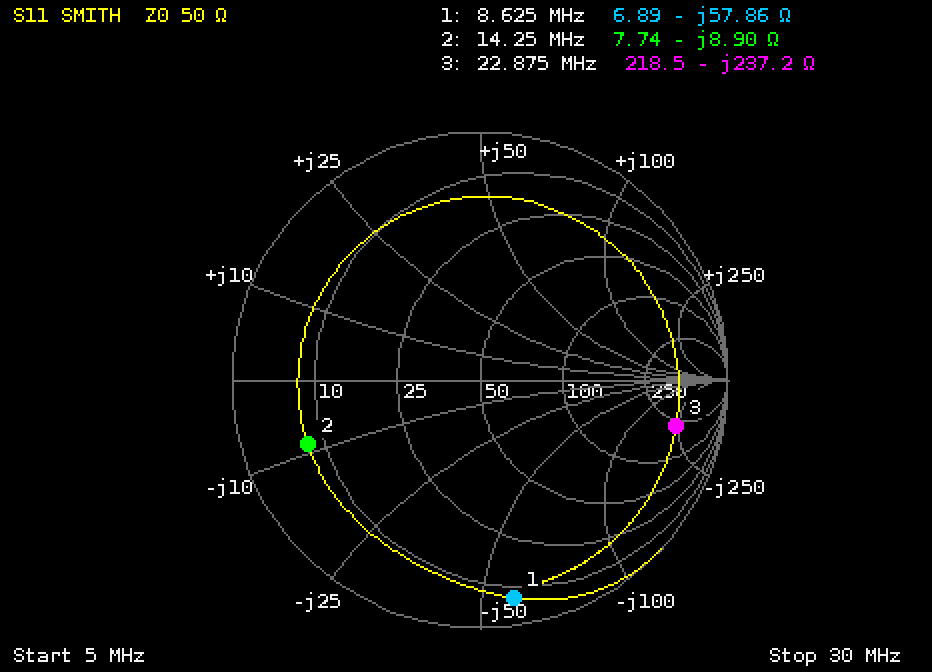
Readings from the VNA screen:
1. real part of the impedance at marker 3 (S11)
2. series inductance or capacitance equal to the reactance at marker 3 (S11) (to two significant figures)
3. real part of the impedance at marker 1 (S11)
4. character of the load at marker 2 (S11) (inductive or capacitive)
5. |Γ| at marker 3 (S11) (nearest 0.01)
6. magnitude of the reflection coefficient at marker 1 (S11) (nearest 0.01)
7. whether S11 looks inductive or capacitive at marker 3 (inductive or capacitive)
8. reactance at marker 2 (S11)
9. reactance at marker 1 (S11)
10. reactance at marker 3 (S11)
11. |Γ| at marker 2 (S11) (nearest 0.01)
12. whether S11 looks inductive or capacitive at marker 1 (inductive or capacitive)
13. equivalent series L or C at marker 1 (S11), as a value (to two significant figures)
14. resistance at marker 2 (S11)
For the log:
218.5 Ω
29 pF
6.89 Ω
capacitive
0.81
0.89
capacitive
-8.90 Ω
-57.86 Ω
-237.2 Ω
0.74
capacitive
320 pF
7.74 Ω
